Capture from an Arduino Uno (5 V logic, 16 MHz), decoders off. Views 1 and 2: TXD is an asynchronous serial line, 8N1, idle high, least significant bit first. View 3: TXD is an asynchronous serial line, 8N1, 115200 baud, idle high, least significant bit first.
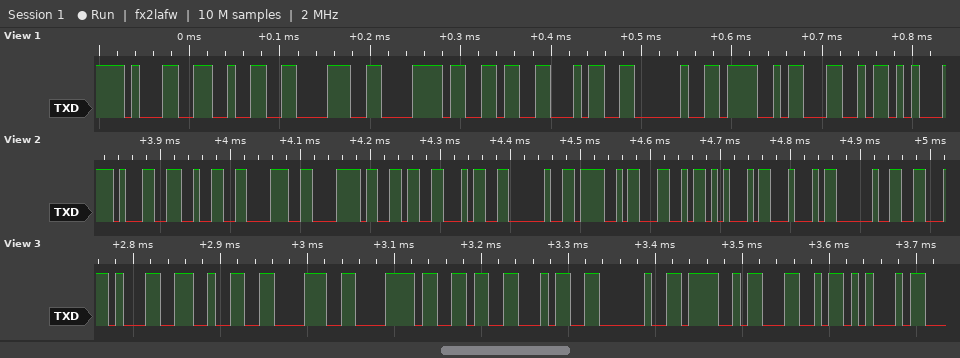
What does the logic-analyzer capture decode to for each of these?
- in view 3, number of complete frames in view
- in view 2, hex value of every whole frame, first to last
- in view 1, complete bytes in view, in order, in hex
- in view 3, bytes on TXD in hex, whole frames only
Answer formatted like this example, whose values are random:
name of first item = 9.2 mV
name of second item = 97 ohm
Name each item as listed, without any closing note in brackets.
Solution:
in view 3, number of complete frames in view = 10
in view 2, hex value of every whole frame, first to last = 31 32 38 78 36 34 20 4F 4C 45 44 20
in view 1, complete bytes in view, in order, in hex = 31 32 38 78 36 34 20 4F 4C
in view 3, bytes on TXD in hex, whole frames only = 0x31 0x32 0x38 0x78 0x36 0x34 0x20 0x4F 0x4C 0x45
